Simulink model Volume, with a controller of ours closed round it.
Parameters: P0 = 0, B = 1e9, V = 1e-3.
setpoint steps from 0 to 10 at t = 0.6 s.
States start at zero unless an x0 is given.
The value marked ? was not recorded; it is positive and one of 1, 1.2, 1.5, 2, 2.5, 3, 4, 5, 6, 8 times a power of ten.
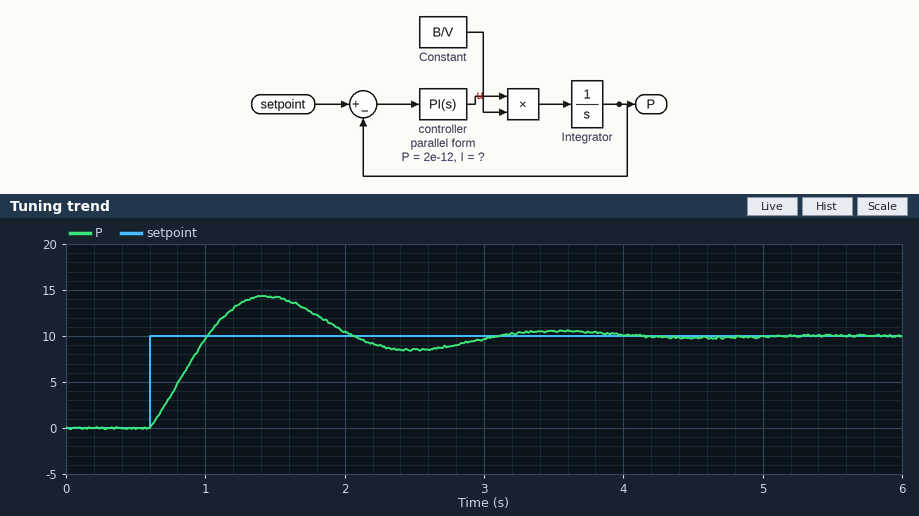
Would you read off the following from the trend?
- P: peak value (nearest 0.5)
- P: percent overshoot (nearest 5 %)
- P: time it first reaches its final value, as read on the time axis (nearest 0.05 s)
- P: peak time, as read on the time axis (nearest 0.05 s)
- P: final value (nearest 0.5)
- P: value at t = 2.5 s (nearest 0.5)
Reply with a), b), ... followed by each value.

a) 14.5
b) 45 %
c) 1.00 s
d) 1.45 s
e) 10.0
f) 8.5
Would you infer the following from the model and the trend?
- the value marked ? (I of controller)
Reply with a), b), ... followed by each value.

a) 1e-11
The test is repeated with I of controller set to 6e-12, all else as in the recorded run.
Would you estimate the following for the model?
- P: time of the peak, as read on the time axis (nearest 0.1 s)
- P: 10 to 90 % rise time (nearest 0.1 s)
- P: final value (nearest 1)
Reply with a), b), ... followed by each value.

a) 1.6 s
b) 0.4 s
c) 10
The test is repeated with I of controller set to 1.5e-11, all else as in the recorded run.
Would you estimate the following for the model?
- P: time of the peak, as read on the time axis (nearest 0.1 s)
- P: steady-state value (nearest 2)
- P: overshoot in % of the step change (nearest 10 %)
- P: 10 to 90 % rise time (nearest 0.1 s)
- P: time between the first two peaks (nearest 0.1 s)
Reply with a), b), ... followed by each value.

a) 1.3 s
b) 10
c) 50 %
d) 0.3 s
e) 1.7 s
